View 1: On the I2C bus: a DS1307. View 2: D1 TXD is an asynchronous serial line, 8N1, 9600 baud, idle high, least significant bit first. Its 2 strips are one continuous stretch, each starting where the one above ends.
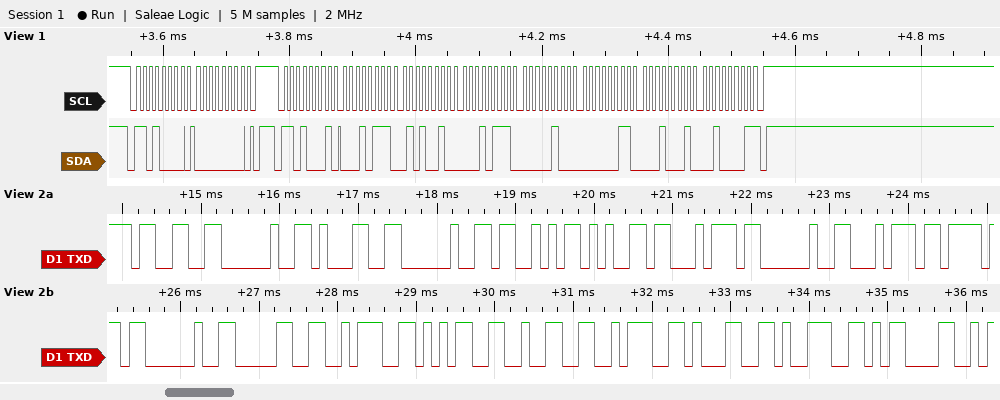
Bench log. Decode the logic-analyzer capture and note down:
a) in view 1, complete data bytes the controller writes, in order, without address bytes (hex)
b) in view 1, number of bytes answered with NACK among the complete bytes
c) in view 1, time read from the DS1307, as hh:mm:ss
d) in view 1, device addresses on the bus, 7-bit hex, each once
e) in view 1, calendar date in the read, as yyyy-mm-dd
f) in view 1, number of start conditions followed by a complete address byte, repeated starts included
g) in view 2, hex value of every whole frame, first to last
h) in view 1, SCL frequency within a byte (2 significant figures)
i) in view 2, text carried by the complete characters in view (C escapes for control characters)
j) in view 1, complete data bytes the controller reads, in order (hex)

00
1
17:52:17
0x68
2021-11-03
2
33 20 31 20 53 65 74 20 74 6F 20 30 3A 35 32 3A 31 39 0D
100 kHz
"3 1 Set to 0:52:19\r"
17 52 17 04 03 11 21
